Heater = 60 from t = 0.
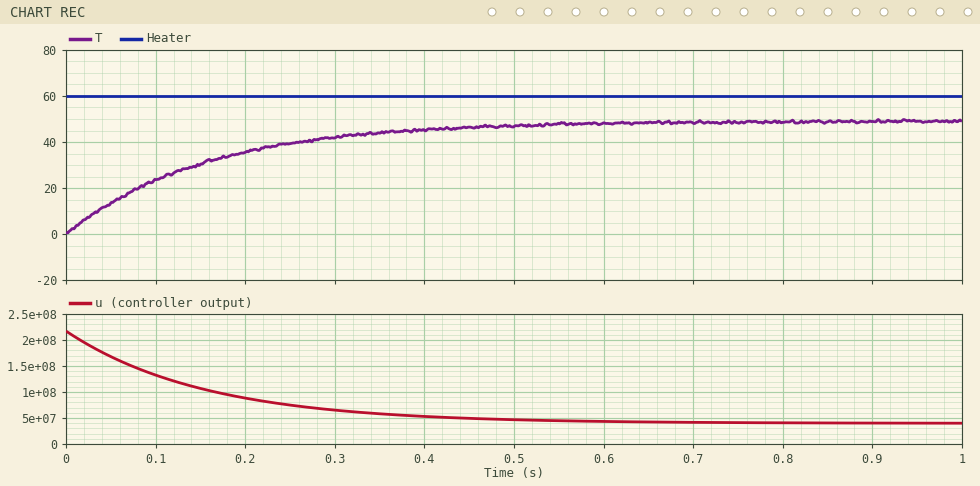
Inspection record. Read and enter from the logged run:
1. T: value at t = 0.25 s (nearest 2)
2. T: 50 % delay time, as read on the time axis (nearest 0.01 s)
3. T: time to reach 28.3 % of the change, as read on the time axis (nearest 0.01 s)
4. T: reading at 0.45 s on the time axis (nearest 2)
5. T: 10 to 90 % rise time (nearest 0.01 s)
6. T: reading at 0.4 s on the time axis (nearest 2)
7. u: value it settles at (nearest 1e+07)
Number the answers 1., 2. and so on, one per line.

1. 40
2. 0.11 s
3. 0.05 s
4. 46
5. 0.34 s
6. 46
7. 40000000
